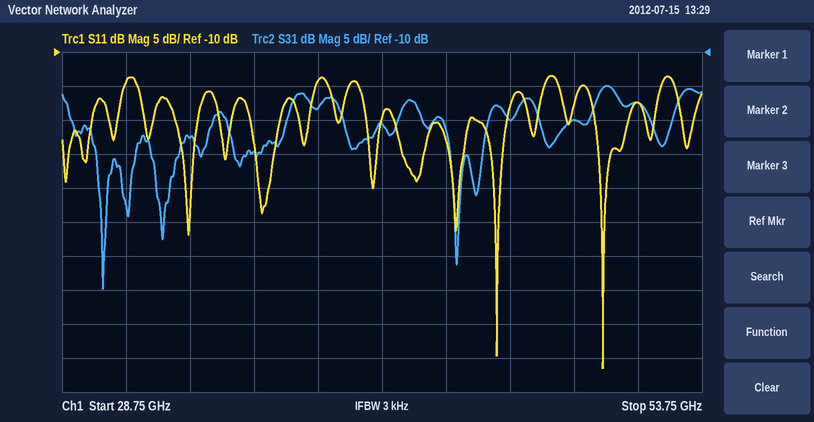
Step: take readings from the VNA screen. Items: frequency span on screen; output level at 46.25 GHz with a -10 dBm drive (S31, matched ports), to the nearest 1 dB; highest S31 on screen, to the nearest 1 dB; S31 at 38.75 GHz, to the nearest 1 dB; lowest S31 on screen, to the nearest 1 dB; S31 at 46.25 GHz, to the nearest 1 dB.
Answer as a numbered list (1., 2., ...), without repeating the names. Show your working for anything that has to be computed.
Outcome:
1. 25 GHz
2. -10 dBm + (-20 dB) = -30 dBm
3. -15 dB
4. -18 dB
5. -45 dB
6. -20 dB
